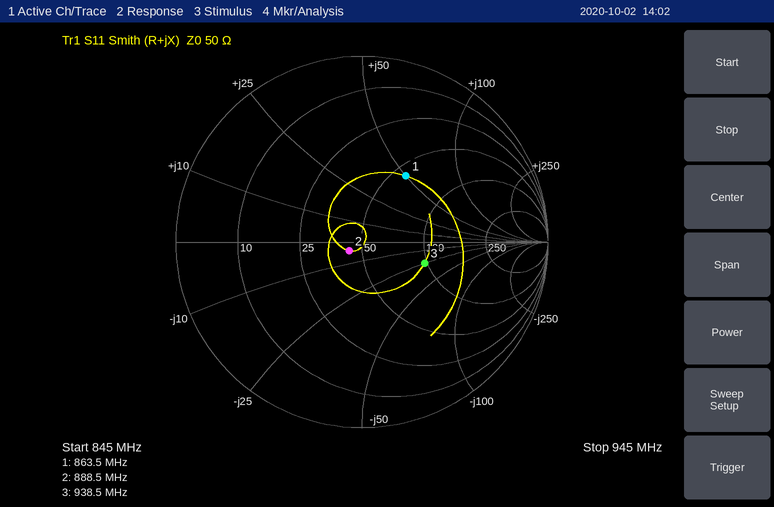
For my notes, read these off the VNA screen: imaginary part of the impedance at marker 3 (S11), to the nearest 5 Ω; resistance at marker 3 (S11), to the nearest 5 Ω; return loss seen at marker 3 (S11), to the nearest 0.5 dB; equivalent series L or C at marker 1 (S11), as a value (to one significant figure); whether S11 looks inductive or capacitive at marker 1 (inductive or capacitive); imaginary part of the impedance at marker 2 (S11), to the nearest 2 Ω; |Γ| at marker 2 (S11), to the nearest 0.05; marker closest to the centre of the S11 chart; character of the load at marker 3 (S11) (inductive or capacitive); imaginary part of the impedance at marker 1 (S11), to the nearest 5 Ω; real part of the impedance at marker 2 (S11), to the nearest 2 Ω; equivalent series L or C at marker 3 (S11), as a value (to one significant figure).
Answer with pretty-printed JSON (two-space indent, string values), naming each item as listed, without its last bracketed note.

{
  "imaginary part of the impedance at marker 3 (S11), to the nearest 5 Ω": "-25 Ω",
  "resistance at marker 3 (S11), to the nearest 5 Ω": "95 Ω",
  "return loss seen at marker 3 (S11), to the nearest 0.5 dB": "9.0 dB",
  "equivalent series L or C at marker 1 (S11), as a value": "9 nH",
  "whether S11 looks inductive or capacitive at marker 1": "inductive",
  "imaginary part of the impedance at marker 2 (S11), to the nearest 2 Ω": "-4 Ω",
  "|Γ| at marker 2 (S11), to the nearest 0.05": "0.10",
  "marker closest to the centre of the S11 chart": "marker 2",
  "character of the load at marker 3 (S11)": "capacitive",
  "imaginary part of the impedance at marker 1 (S11), to the nearest 5 Ω": "+50 Ω",
  "real part of the impedance at marker 2 (S11), to the nearest 2 Ω": "44 Ω",
  "equivalent series L or C at marker 3 (S11), as a value": "7 pF"
}
